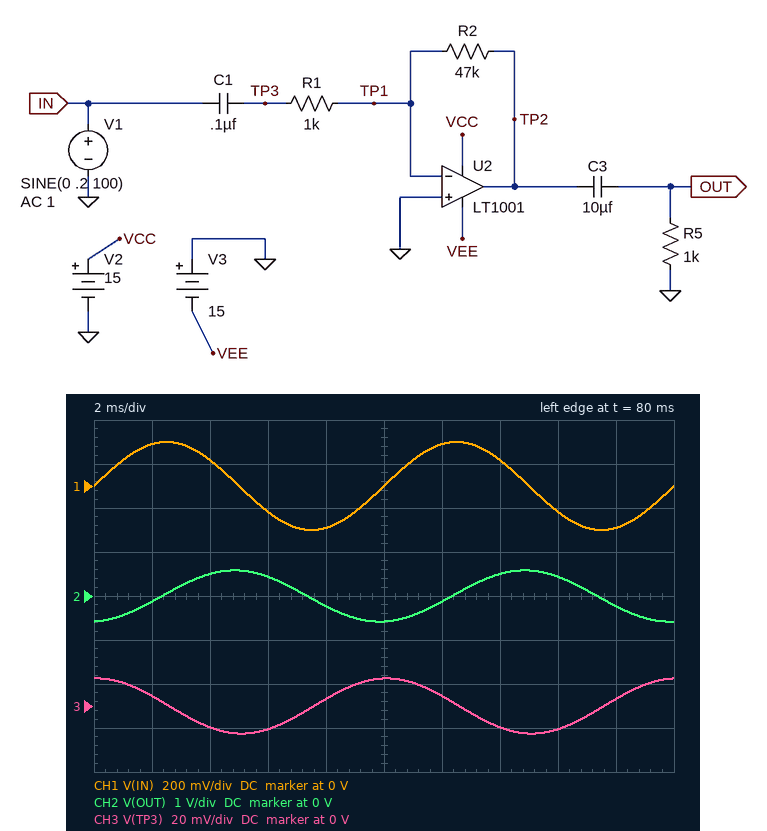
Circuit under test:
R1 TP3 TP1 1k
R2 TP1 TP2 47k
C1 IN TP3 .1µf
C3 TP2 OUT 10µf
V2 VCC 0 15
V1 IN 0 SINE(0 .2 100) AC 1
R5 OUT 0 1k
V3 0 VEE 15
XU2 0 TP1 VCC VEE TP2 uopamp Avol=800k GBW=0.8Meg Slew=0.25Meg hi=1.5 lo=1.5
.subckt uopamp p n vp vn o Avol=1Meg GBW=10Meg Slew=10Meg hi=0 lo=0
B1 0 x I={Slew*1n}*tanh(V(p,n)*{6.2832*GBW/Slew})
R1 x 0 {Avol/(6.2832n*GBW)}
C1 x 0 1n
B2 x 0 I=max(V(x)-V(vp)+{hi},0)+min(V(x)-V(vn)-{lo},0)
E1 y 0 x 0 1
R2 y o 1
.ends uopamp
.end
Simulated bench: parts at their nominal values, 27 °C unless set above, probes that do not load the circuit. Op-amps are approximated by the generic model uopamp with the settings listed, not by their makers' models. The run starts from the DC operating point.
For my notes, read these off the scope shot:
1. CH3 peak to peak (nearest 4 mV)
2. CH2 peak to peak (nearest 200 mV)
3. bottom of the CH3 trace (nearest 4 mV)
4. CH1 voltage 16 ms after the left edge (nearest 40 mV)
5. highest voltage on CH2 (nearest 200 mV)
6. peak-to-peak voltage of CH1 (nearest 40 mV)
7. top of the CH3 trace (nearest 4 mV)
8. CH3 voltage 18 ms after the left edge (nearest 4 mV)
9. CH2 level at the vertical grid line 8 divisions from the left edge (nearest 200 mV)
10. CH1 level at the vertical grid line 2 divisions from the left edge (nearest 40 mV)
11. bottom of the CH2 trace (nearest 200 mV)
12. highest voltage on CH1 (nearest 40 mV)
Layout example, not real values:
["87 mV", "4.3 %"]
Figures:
["24 mV", "1.2 V", "-12 mV", "-120 mV", "600 mV", "400 mV", "12 mV", "4 mV", "400 mV", "120 mV", "-600 mV", "200 mV"]
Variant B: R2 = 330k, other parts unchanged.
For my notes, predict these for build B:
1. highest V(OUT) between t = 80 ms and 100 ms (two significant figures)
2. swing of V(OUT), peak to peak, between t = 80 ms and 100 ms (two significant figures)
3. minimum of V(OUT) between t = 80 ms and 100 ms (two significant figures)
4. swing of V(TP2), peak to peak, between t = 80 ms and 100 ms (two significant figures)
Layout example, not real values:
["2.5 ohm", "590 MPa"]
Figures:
["4.1 V", "8.2 V", "-4.1 V", "8.3 V"]
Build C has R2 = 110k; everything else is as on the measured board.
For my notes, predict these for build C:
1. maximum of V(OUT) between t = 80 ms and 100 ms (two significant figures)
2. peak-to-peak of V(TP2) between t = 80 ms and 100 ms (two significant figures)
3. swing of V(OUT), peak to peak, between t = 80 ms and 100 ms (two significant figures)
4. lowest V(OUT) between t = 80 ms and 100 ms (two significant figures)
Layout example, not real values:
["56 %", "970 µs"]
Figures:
["1.4 V", "2.8 V", "2.7 V", "-1.4 V"]
